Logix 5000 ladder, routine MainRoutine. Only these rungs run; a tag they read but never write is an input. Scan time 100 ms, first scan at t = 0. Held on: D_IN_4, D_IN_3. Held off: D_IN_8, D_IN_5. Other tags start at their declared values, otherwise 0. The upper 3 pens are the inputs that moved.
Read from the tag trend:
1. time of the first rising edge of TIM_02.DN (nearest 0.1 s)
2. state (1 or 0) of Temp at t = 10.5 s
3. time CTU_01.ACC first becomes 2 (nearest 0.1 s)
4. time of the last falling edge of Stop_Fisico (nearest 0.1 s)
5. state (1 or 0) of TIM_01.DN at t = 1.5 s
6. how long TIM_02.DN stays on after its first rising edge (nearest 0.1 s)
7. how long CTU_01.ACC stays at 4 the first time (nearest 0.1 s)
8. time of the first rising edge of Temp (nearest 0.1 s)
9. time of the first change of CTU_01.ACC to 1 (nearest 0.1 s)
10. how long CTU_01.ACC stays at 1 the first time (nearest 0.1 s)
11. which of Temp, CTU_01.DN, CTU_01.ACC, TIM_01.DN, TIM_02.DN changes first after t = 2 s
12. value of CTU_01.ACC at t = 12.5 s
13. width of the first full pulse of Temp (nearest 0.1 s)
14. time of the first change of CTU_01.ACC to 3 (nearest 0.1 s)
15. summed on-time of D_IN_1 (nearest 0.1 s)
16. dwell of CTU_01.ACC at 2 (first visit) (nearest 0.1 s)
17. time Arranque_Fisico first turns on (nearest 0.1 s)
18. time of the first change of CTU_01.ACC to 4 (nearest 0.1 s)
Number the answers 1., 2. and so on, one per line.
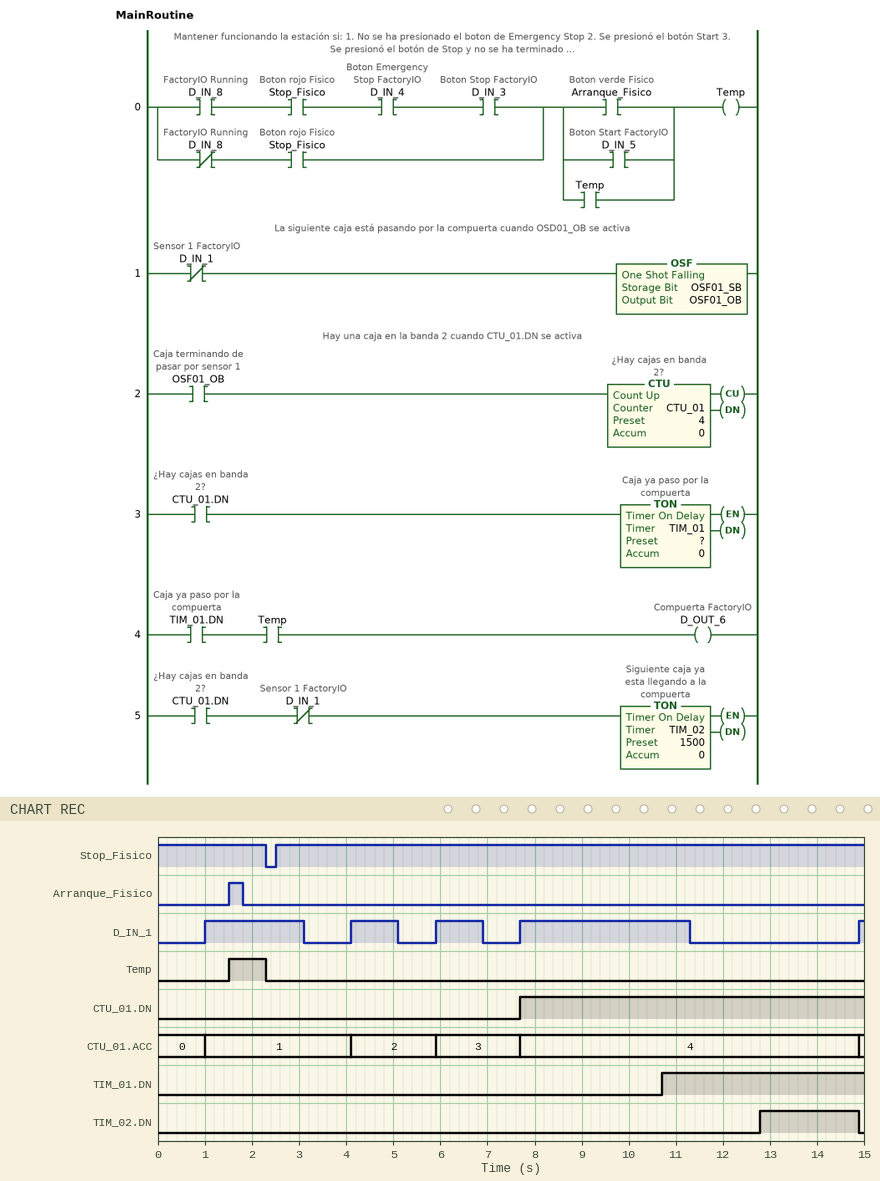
1. 12.8 s
2. 0
3. 4.1 s
4. 2.3 s
5. 0
6. 2.1 s
7. 7.2 s
8. 1.5 s
9. 1.0 s
10. 3.1 s
11. Temp
12. 4
13. 0.8 s
14. 5.9 s
15. 7.8 s
16. 1.8 s
17. 1.5 s
18. 7.7 s
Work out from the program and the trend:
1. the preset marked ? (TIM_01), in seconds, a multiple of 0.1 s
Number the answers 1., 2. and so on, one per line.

1. 3.0 s
